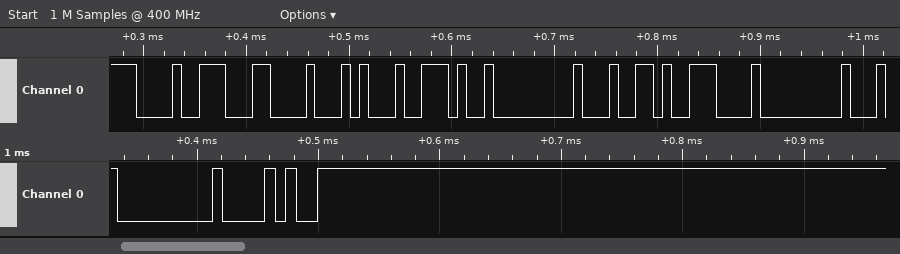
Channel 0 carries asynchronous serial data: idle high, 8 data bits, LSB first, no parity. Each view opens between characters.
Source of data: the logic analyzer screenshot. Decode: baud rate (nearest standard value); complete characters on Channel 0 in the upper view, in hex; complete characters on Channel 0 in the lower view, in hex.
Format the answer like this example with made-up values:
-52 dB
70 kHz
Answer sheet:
115200 baud
C8, 0C, 14, 2E, 00, 64, 0E, 00
00, 28
